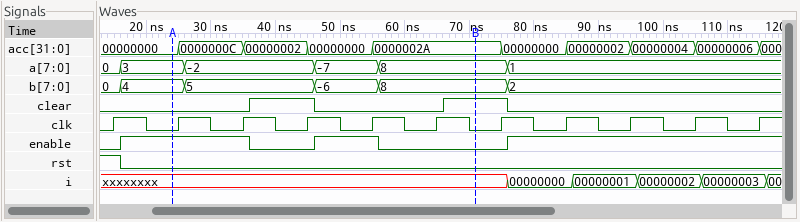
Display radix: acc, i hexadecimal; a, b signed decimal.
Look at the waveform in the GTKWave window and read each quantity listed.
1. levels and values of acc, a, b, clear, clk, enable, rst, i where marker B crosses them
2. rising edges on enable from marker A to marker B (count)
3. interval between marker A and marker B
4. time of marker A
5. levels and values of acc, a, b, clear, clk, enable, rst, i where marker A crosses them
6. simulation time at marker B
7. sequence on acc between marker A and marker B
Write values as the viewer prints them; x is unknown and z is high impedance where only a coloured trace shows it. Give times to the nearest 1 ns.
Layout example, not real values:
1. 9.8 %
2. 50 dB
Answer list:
1. acc=0000002A, a=8, b=8, clear=1, clk=0, enable=0, rst=0, i=xxxxxxxx
2. 1
3. 47 ns
4. 24 ns
5. acc=00000000, a=3, b=4, clear=0, clk=0, enable=1, rst=0, i=xxxxxxxx
6. 71 ns
7. 00000000, 0000000C, 00000002, 00000000, 0000002A
